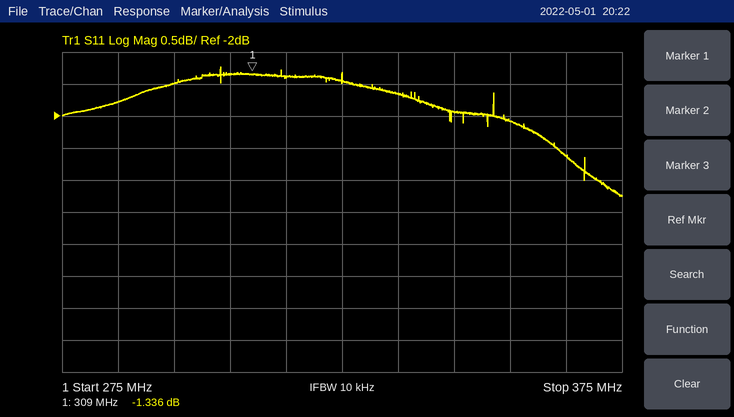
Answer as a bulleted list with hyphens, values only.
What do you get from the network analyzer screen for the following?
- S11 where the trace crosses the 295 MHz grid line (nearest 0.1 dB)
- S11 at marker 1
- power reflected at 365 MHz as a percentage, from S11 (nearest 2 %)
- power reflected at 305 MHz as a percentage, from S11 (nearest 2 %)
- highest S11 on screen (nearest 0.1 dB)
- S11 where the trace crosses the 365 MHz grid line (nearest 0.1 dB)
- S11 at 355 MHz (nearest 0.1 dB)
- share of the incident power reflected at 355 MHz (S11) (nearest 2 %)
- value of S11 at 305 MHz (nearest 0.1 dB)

- -1.5 dB
- -1.336 dB
- 54 %
- 74 %
- -1.2 dB
- -2.6 dB
- -2.1 dB
- 62 %
- -1.3 dB
